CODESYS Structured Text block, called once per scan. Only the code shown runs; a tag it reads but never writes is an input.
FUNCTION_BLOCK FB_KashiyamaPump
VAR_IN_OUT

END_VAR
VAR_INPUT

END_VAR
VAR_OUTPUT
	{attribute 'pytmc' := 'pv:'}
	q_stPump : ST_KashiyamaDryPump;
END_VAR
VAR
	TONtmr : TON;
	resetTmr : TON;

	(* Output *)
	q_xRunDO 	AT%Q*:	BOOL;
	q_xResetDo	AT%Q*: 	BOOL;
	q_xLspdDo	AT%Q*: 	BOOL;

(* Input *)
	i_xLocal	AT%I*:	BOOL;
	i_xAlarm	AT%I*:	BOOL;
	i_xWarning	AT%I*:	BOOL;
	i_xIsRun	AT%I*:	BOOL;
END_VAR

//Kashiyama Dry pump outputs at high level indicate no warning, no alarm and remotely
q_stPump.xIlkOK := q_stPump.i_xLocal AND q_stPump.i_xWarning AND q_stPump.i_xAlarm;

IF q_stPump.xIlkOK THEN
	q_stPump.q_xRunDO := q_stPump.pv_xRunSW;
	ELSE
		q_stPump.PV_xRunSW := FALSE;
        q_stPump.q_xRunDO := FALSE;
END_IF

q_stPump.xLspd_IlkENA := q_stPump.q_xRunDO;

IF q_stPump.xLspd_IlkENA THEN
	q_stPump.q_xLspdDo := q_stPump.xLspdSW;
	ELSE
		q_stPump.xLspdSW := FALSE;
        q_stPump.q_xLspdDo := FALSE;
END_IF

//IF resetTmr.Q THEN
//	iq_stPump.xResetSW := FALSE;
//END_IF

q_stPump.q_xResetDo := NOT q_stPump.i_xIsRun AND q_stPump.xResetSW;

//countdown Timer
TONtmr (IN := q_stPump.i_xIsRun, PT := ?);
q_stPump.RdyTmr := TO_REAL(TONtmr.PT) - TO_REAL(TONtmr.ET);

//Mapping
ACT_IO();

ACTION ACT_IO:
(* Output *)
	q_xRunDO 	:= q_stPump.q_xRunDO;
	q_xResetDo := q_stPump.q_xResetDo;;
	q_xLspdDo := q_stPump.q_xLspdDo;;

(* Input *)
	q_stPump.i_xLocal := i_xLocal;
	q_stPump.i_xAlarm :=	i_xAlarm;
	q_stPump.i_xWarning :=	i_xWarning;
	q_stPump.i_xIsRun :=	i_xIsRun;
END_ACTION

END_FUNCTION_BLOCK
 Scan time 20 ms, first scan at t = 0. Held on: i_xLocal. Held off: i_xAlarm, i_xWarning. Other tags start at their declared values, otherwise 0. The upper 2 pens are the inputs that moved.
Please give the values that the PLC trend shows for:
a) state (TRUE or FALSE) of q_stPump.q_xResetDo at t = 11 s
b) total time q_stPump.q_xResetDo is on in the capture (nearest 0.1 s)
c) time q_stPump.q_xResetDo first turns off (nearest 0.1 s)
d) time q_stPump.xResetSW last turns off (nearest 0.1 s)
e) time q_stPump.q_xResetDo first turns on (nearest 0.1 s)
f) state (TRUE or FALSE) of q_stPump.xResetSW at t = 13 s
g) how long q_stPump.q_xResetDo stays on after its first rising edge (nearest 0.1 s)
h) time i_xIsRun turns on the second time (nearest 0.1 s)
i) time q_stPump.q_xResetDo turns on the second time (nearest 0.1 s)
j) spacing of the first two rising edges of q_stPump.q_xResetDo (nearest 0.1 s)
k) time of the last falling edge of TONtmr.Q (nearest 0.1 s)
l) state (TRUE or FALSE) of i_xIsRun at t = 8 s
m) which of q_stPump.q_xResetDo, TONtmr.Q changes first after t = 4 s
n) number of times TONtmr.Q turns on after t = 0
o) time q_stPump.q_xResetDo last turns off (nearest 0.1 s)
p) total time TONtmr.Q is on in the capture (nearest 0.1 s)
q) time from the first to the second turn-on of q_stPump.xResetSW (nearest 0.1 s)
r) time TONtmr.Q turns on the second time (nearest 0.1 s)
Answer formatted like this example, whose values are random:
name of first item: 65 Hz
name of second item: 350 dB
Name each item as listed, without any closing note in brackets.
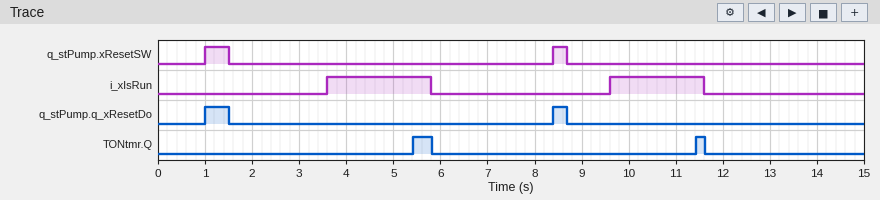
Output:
state (TRUE or FALSE) of q_stPump.q_xResetDo at t = 11 s: FALSE
total time q_stPump.q_xResetDo is on in the capture: 0.8 s
time q_stPump.q_xResetDo first turns off: 1.5 s
time q_stPump.xResetSW last turns off: 8.7 s
time q_stPump.q_xResetDo first turns on: 1.0 s
state (TRUE or FALSE) of q_stPump.xResetSW at t = 13 s: FALSE
how long q_stPump.q_xResetDo stays on after its first rising edge: 0.5 s
time i_xIsRun turns on the second time: 9.6 s
time q_stPump.q_xResetDo turns on the second time: 8.4 s
spacing of the first two rising edges of q_stPump.q_xResetDo: 7.4 s
time of the last falling edge of TONtmr.Q: 11.6 s
state (TRUE or FALSE) of i_xIsRun at t = 8 s: FALSE
which of q_stPump.q_xResetDo, TONtmr.Q changes first after t = 4 s: TONtmr.Q
number of times TONtmr.Q turns on after t = 0: 2
time q_stPump.q_xResetDo last turns off: 8.7 s
total time TONtmr.Q is on in the capture: 0.6 s
time from the first to the second turn-on of q_stPump.xResetSW: 7.4 s
time TONtmr.Q turns on the second time: 11.4 s
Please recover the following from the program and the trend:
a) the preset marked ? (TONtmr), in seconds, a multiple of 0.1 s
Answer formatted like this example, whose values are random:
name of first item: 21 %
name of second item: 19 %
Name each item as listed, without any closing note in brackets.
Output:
the preset marked ? (TONtmr), in seconds, a multiple of 0.1 s: 1.8 s
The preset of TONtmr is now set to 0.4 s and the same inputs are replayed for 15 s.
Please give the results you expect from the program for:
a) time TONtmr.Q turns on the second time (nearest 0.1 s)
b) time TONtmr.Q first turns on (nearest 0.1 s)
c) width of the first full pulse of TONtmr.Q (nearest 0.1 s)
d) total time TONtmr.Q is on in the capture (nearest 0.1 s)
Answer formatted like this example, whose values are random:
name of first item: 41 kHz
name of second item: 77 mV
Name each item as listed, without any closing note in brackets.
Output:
time TONtmr.Q turns on the second time: 10.0 s
time TONtmr.Q first turns on: 4.0 s
width of the first full pulse of TONtmr.Q: 1.8 s
total time TONtmr.Q is on in the capture: 3.4 s
